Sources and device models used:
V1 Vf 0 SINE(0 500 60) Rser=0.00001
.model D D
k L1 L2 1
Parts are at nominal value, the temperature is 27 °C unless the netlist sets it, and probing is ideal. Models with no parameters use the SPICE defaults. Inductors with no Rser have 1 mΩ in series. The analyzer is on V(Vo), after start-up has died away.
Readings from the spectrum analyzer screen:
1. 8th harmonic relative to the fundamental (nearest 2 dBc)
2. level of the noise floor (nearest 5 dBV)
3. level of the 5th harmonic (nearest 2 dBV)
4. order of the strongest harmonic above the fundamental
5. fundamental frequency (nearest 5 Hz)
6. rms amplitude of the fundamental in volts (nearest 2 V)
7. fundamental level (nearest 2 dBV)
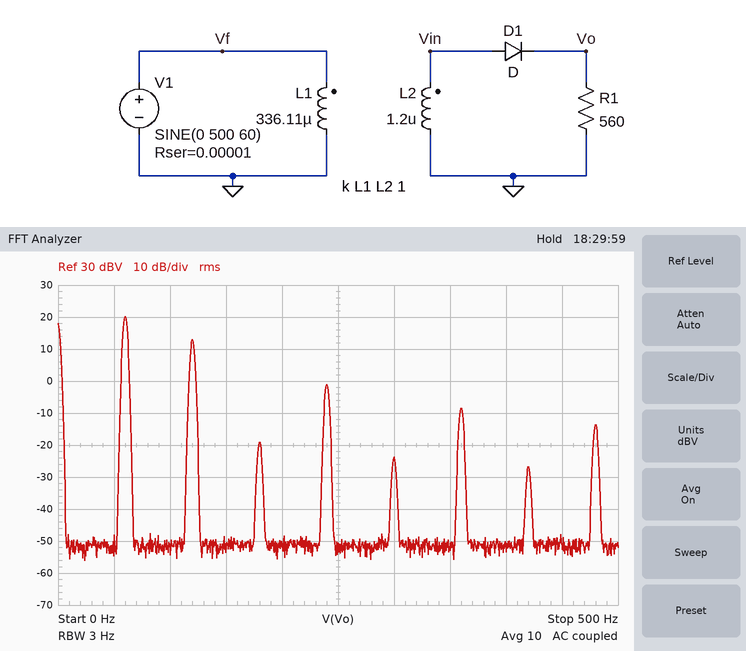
-34 dBc
-50 dBV
-24 dBV
2
60 Hz
10 V
20 dBV
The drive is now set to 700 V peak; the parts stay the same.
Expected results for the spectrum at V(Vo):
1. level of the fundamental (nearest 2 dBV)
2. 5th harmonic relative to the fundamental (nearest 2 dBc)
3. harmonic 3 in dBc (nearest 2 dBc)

24 dBV
-46 dBc
-42 dBc
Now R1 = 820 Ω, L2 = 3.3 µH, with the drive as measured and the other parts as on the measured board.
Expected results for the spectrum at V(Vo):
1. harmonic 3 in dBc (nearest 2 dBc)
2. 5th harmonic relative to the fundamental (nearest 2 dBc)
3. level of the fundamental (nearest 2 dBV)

-44 dBc
-48 dBc
24 dBV
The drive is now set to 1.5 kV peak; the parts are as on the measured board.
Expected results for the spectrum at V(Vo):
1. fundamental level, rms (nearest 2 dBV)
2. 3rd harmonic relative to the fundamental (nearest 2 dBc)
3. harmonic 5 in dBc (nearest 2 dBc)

30 dBV
-48 dBc
-52 dBc
